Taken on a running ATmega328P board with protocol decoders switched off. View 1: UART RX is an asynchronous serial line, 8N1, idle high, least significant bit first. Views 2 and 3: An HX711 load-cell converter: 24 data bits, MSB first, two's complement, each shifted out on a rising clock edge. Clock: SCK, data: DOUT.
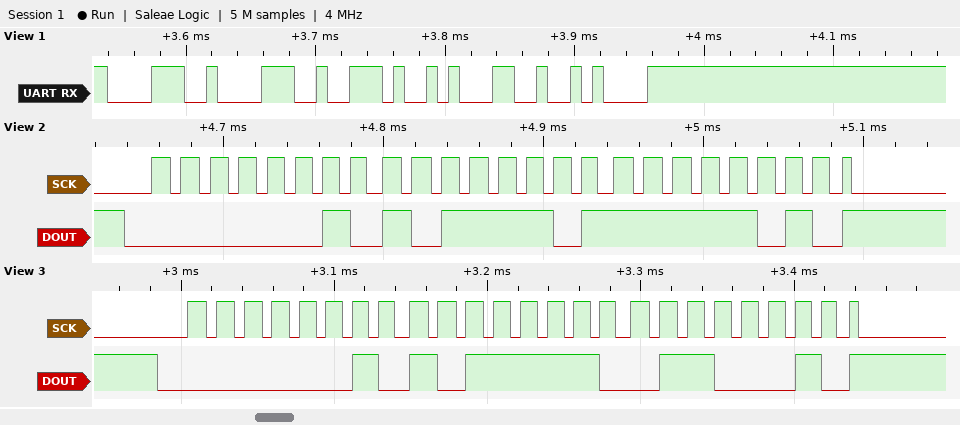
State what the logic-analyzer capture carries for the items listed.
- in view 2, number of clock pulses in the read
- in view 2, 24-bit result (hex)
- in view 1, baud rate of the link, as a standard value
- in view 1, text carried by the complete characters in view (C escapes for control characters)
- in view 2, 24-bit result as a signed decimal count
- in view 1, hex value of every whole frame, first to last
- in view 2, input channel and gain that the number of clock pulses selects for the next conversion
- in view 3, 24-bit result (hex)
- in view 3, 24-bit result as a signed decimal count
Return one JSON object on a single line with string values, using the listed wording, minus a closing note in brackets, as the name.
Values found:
{"in view 2, number of clock pulses in the read": "25", "in view 2, 24-bit result": "0x02BDFA", "in view 1, baud rate of the link, as a standard value": "115200 baud", "in view 1, text carried by the complete characters in view": "\"88.1\\n\"", "in view 2, 24-bit result as a signed decimal count": "179706", "in view 1, hex value of every whole frame, first to last": "38 38 2E 31 0A", "in view 2, input channel and gain that the number of clock pulses selects for the next conversion": "channel A, gain 128", "in view 3, 24-bit result": "0x02BE62", "in view 3, 24-bit result as a signed decimal count": "179810"}
